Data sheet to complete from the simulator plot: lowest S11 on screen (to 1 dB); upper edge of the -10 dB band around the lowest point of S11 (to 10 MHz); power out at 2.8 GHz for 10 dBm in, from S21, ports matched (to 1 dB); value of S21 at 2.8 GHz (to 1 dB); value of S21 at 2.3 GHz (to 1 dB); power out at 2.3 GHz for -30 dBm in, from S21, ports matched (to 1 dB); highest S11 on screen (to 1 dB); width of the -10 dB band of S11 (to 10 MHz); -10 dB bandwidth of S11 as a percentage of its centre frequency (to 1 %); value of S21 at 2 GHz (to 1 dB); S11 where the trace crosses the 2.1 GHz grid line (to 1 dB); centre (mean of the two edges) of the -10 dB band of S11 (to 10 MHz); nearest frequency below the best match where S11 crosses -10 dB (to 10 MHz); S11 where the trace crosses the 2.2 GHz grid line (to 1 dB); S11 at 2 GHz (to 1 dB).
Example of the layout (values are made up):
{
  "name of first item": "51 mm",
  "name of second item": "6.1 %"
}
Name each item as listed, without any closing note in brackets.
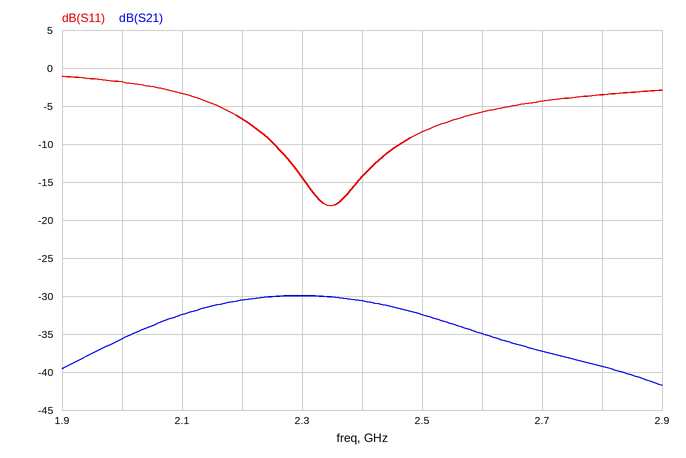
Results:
{
  "lowest S11 on screen": "-18 dB",
  "upper edge of the -10 dB band around the lowest point of S11": "2.46 GHz",
  "power out at 2.8 GHz for 10 dBm in, from S21, ports matched": "-29 dBm",
  "value of S21 at 2.8 GHz": "-39 dB",
  "value of S21 at 2.3 GHz": "-30 dB",
  "power out at 2.3 GHz for -30 dBm in, from S21, ports matched": "-60 dBm",
  "highest S11 on screen": "-1 dB",
  "width of the -10 dB band of S11": "210 MHz",
  "-10 dB bandwidth of S11 as a percentage of its centre frequency": "9 %",
  "value of S21 at 2 GHz": "-36 dB",
  "S11 where the trace crosses the 2.1 GHz grid line": "-3 dB",
  "centre (mean of the two edges) of the -10 dB band of S11": "2.36 GHz",
  "nearest frequency below the best match where S11 crosses -10 dB": "2.25 GHz",
  "S11 where the trace crosses the 2.2 GHz grid line": "-7 dB",
  "S11 at 2 GHz": "-2 dB"
}
